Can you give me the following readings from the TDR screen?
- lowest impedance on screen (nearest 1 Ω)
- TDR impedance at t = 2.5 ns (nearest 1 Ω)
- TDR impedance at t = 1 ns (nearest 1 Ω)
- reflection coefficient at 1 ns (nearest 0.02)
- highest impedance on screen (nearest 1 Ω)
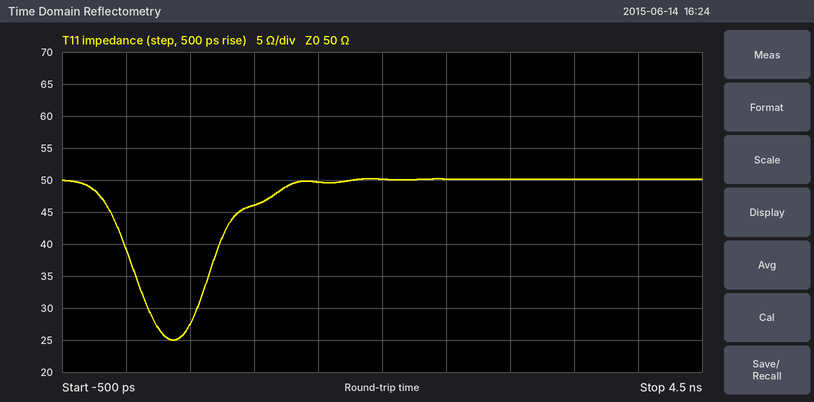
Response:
25 Ω
50 Ω
46 Ω
-0.04
50 Ω
